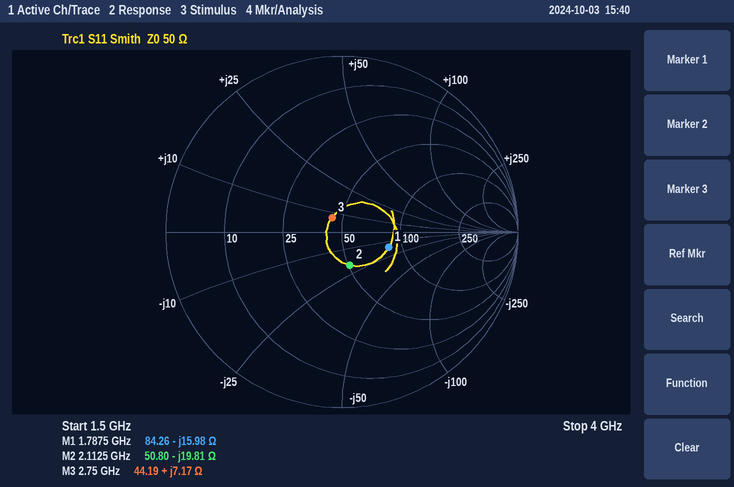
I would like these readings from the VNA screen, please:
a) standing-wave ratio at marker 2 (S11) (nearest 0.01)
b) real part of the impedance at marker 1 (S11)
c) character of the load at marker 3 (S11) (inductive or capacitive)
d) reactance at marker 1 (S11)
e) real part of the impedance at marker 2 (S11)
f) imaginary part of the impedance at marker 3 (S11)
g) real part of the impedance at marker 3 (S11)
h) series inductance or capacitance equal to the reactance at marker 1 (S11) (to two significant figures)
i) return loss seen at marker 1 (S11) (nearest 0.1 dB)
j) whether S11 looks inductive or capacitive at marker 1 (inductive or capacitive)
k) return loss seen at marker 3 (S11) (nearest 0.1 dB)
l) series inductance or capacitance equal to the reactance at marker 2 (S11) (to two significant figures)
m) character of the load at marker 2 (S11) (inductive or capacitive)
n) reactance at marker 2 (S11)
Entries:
1.48
84.26 Ω
inductive
-15.98 Ω
50.80 Ω
+7.17 Ω
44.19 Ω
5.6 pF
11.1 dB
capacitive
20.2 dB
3.8 pF
capacitive
-19.81 Ω
